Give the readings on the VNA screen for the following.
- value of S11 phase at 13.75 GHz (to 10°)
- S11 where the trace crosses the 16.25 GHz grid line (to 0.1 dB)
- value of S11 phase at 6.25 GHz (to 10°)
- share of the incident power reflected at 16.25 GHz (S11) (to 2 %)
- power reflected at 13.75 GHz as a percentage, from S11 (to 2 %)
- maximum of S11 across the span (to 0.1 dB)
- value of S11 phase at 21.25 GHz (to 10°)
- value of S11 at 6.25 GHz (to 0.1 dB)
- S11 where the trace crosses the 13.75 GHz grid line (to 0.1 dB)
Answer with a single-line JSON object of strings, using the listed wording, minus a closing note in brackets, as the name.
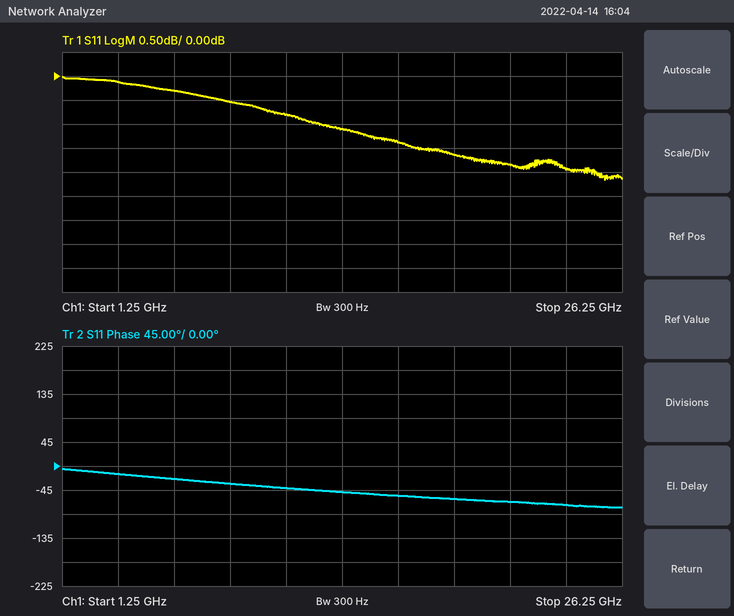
{"value of S11 phase at 13.75 GHz": "-50°", "S11 where the trace crosses the 16.25 GHz grid line": "-1.4 dB", "value of S11 phase at 6.25 GHz": "-20°", "share of the incident power reflected at 16.25 GHz (S11)": "72 %", "power reflected at 13.75 GHz as a percentage, from S11": "78 %", "maximum of S11 across the span": "0.0 dB", "value of S11 phase at 21.25 GHz": "-70°", "value of S11 at 6.25 GHz": "-0.3 dB", "S11 where the trace crosses the 13.75 GHz grid line": "-1.1 dB"}
